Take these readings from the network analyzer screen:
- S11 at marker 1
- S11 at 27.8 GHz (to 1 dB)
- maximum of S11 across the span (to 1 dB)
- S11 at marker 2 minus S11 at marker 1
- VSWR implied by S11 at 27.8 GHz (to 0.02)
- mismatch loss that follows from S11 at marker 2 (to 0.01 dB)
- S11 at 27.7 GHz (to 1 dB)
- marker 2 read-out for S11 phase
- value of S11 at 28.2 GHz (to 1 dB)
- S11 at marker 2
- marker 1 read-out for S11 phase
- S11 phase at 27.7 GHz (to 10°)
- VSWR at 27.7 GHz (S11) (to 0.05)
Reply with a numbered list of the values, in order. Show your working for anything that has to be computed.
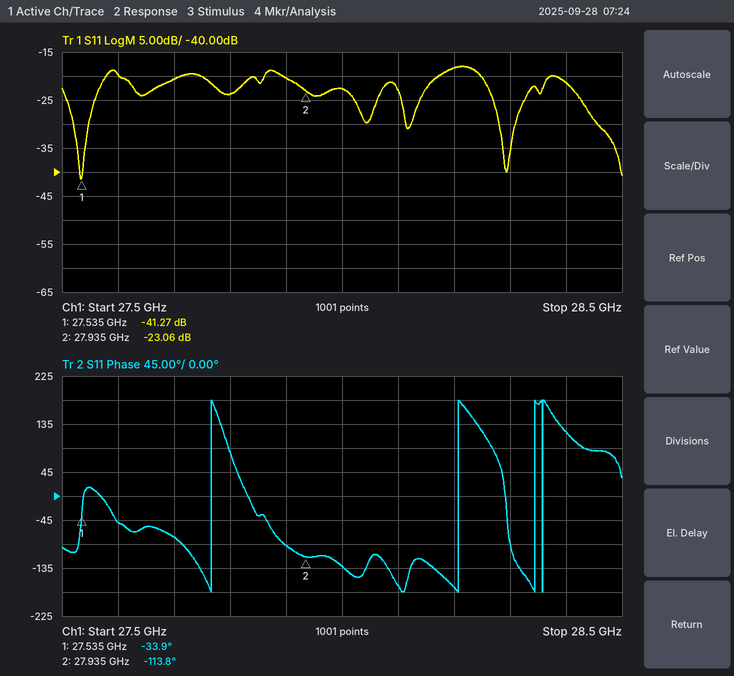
1. -41.27 dB
2. -24 dB
3. -18 dB
4. -23.06 − (-41.27) = 18.21 dB
5. |Γ| = 10^(-24/20) = 0.0631; VSWR = (1 + 0.0631)/(1 − 0.0631) ≈ 1.13, so 1.14 to the nearest 0.02
6. −10 log10(1 − 10^(-23.06/10)) ≈ 0.02 dB
7. -21 dB
8. -113.8°
9. -18 dB
10. -23.06 dB
11. -33.9°
12. -80°
13. |Γ| = 10^(-21/20) = 0.0891; VSWR = (1 + 0.0891)/(1 − 0.0891) ≈ 1.20
